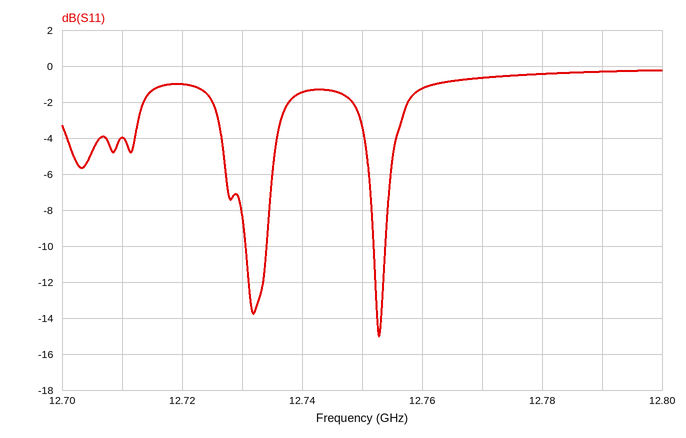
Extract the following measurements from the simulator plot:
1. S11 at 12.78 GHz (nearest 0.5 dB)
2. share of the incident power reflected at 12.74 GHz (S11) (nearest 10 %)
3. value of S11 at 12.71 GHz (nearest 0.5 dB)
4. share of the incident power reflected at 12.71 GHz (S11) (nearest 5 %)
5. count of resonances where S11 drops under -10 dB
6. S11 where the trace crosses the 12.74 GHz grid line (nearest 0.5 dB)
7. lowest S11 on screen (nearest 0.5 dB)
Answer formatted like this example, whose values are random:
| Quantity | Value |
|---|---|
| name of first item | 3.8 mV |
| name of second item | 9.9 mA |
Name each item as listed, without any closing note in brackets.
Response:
| Quantity | Value |
|---|---|
| S11 at 12.78 GHz | -0.5 dB |
| share of the incident power reflected at 12.74 GHz (S11) | 70 % |
| value of S11 at 12.71 GHz | -4.0 dB |
| share of the incident power reflected at 12.71 GHz (S11) | 40 % |
| count of resonances where S11 drops under -10 dB | 2 |
| S11 where the trace crosses the 12.74 GHz grid line | -1.5 dB |
| lowest S11 on screen | -15.0 dB |
